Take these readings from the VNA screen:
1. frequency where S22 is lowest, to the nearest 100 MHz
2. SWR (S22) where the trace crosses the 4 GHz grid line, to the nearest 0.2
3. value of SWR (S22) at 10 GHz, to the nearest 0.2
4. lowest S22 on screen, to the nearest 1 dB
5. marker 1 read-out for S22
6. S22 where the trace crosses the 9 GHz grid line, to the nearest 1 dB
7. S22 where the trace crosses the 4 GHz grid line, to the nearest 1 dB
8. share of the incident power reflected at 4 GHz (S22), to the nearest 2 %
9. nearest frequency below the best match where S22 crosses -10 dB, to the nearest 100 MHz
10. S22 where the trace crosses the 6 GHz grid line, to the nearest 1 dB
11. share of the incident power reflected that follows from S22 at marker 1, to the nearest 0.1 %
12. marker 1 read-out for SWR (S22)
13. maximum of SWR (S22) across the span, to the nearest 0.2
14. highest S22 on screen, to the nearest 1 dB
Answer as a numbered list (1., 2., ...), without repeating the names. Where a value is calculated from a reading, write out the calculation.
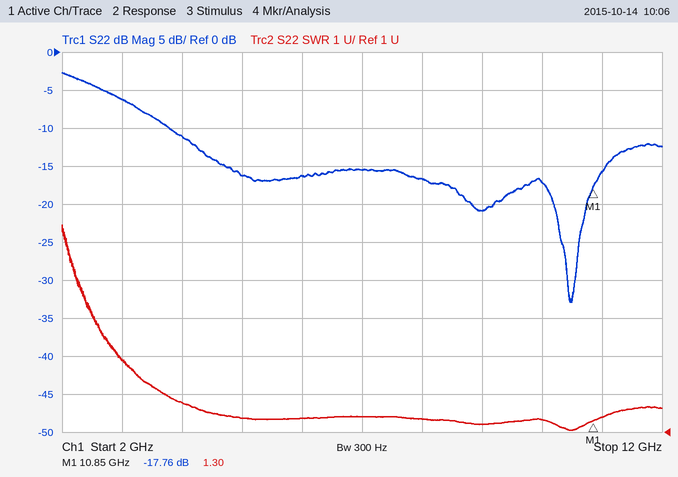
1. 10.5 GHz
2. 1.8
3. 1.4
4. -33 dB
5. -17.76 dB
6. -21 dB
7. -11 dB
8. 10^(-11/10) ≈ 8 %
9. 3.8 GHz
10. -16 dB
11. 10^(-17.76/10) ≈ 1.7 %
12. 1.30
13. 6.4
14. -3 dB
